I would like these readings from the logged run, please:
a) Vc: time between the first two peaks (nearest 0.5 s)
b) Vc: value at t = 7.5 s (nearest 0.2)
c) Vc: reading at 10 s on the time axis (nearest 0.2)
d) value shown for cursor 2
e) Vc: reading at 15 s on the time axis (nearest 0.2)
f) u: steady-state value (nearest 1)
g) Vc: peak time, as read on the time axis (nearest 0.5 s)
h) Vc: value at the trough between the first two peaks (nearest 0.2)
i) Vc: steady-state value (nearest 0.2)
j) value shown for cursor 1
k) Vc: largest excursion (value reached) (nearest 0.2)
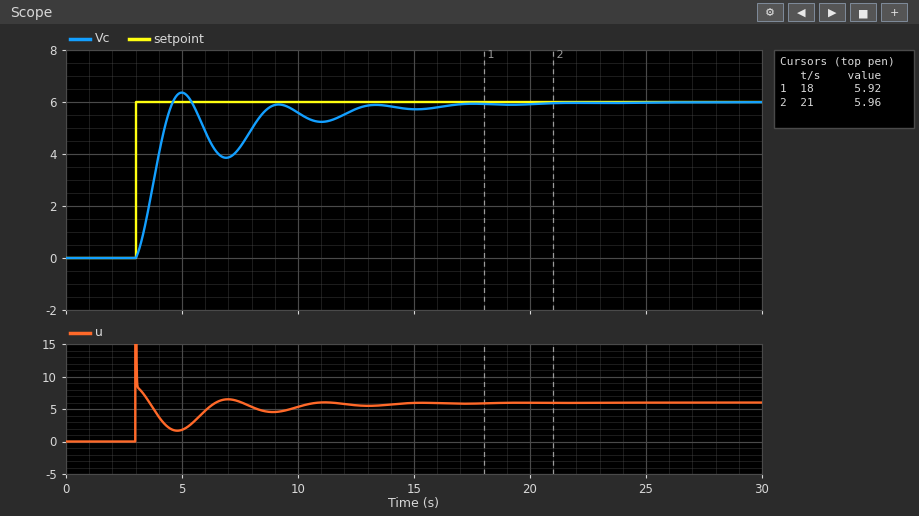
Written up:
4.0 s
4.2
5.6
5.96
5.8
6
5.0 s
3.8
6.0
5.92
6.4
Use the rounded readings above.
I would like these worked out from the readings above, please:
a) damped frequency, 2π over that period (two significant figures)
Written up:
1.6 rad/s
